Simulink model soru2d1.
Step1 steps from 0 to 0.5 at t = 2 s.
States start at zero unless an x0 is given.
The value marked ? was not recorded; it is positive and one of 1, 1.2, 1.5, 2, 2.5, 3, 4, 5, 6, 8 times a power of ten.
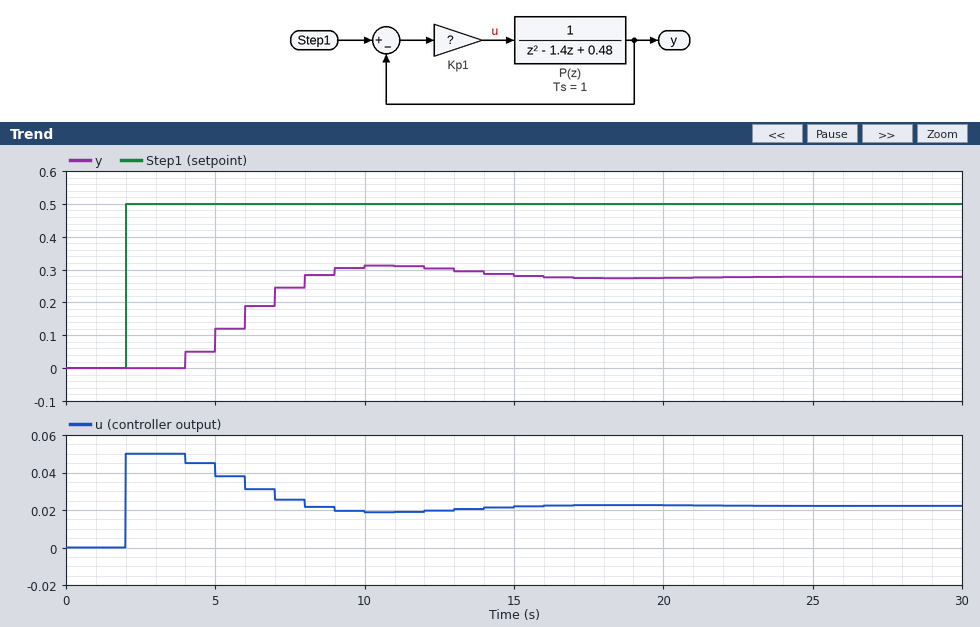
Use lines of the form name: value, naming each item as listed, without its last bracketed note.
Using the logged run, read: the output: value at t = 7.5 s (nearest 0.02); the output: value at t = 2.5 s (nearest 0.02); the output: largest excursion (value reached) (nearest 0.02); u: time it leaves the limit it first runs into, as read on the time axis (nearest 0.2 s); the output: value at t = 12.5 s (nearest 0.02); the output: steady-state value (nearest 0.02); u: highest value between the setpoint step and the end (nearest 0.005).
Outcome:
the output: value at t = 7.5 s: 0.24
the output: value at t = 2.5 s: 0.00
the output: largest excursion (value reached): 0.32
u: time it leaves the limit it first runs into, as read on the time axis: 4.0 s
the output: value at t = 12.5 s: 0.30
the output: steady-state value: 0.28
u: highest value between the setpoint step and the end: 0.050
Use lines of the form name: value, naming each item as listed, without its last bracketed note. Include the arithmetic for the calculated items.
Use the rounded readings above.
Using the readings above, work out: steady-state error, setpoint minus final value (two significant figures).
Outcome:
steady-state error, setpoint minus final value: 0.5 - 0.28 = 0.22
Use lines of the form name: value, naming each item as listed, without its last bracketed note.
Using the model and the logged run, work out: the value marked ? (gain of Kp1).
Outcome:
the value marked ?: 0.1
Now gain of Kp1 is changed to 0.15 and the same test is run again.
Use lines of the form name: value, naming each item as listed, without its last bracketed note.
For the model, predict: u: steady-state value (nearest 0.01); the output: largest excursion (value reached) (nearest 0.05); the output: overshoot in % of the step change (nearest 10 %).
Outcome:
u: steady-state value: 0.03
the output: largest excursion (value reached): 0.40
the output: overshoot in % of the step change: 20 %
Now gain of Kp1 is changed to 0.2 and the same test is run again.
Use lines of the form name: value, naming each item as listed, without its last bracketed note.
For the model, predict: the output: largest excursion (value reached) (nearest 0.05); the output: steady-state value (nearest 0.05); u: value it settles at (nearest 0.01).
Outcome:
the output: largest excursion (value reached): 0.50
the output: steady-state value: 0.35
u: value it settles at: 0.03
